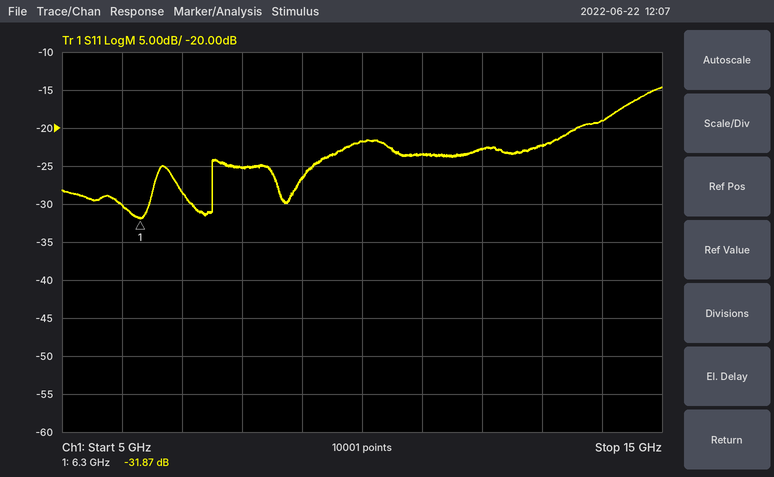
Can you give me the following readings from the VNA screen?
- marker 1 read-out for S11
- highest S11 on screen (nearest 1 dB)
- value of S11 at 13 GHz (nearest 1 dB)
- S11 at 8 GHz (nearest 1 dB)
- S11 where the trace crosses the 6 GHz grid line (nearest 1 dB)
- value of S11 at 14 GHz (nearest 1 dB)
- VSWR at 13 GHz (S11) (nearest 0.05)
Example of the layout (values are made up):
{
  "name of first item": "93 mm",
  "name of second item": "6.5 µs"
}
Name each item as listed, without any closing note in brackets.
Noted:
{
  "marker 1 read-out for S11": "-31.87 dB",
  "highest S11 on screen": "-15 dB",
  "value of S11 at 13 GHz": "-22 dB",
  "S11 at 8 GHz": "-25 dB",
  "S11 where the trace crosses the 6 GHz grid line": "-30 dB",
  "value of S11 at 14 GHz": "-19 dB",
  "VSWR at 13 GHz (S11)": "1.15"
}
